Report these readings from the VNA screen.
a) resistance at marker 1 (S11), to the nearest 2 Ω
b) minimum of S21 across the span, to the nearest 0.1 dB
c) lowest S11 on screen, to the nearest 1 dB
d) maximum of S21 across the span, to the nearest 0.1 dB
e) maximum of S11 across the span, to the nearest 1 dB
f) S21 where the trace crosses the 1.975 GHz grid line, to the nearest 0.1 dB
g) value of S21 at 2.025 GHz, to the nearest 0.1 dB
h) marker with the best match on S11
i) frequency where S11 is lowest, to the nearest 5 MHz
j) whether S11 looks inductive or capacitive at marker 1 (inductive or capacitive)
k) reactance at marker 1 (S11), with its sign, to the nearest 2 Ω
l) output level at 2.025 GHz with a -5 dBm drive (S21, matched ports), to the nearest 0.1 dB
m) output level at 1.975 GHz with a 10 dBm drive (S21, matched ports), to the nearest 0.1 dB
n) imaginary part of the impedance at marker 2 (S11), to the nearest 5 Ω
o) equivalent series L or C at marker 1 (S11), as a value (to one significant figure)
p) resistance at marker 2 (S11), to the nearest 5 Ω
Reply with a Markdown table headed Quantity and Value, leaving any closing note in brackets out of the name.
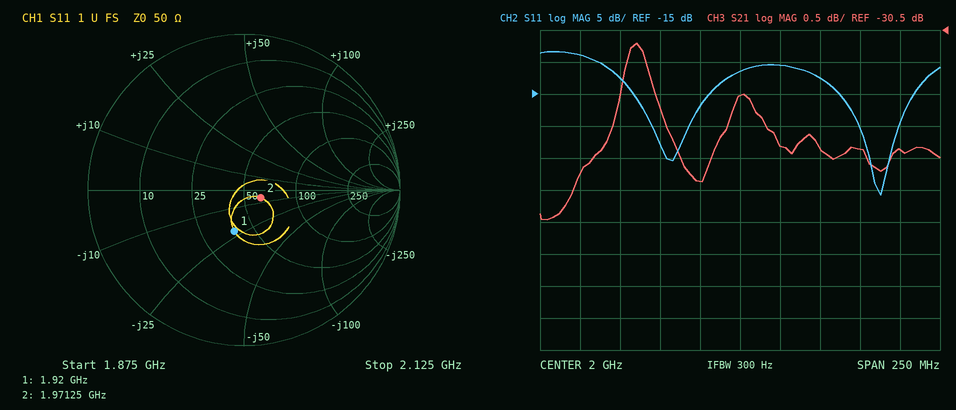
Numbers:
| Quantity | Value |
|---|---|
| resistance at marker 1 (S11), to the nearest 2 Ω | 38 Ω |
| minimum of S21 across the span, to the nearest 0.1 dB | -33.5 dB |
| lowest S11 on screen, to the nearest 1 dB | -31 dB |
| maximum of S21 across the span, to the nearest 0.1 dB | -30.7 dB |
| maximum of S11 across the span, to the nearest 1 dB | -8 dB |
| S21 where the trace crosses the 1.975 GHz grid line, to the nearest 0.1 dB | -32.9 dB |
| value of S21 at 2.025 GHz, to the nearest 0.1 dB | -32.3 dB |
| marker with the best match on S11 | marker 2 |
| frequency where S11 is lowest, to the nearest 5 MHz | 2.090 GHz |
| whether S11 looks inductive or capacitive at marker 1 | capacitive |
| reactance at marker 1 (S11), with its sign, to the nearest 2 Ω | -22 Ω |
| output level at 2.025 GHz with a -5 dBm drive (S21, matched ports), to the nearest 0.1 dB | -37.3 dBm |
| output level at 1.975 GHz with a 10 dBm drive (S21, matched ports), to the nearest 0.1 dB | -22.9 dBm |
| imaginary part of the impedance at marker 2 (S11), to the nearest 5 Ω | -5 Ω |
| equivalent series L or C at marker 1 (S11), as a value | 4 pF |
| resistance at marker 2 (S11), to the nearest 5 Ω | 60 Ω |
